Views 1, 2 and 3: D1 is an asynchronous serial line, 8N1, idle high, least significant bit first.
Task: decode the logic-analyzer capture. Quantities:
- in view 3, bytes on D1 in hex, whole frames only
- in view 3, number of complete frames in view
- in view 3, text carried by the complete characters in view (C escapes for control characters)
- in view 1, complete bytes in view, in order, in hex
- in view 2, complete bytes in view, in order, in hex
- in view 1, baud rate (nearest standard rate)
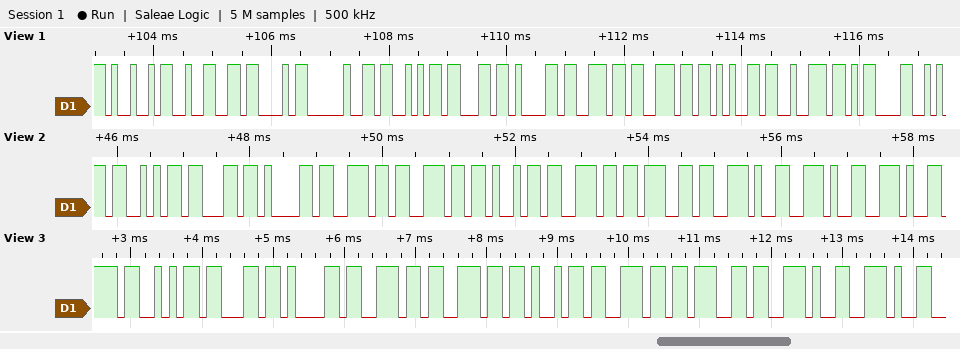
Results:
0x53 0x63 0x61 0x6E 0x6E 0x69 0x6E 0x67 0x2E 0x2E
10
"Scanning.."
49 32 43 20 53 63 61 6E 6E 65 72 0D
53 63 61 6E 6E 69 6E 67 2E 2E 2E
9600 baud
